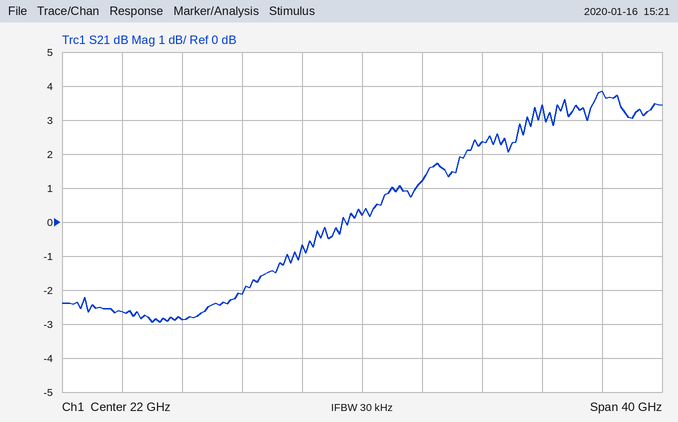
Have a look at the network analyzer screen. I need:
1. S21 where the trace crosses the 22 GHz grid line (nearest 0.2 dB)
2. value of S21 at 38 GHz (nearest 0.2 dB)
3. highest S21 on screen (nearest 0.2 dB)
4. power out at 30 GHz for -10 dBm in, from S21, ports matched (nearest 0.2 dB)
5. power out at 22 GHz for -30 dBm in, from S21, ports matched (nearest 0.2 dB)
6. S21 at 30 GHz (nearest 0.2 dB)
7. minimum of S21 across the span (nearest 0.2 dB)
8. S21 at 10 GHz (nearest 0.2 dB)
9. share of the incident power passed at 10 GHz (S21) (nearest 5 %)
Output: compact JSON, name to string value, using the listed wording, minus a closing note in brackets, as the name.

{"S21 where the trace crosses the 22 GHz grid line": "0.2 dB", "value of S21 at 38 GHz": "3.8 dB", "highest S21 on screen": "3.8 dB", "power out at 30 GHz for -10 dBm in, from S21, ports matched": "-7.6 dBm", "power out at 22 GHz for -30 dBm in, from S21, ports matched": "-29.8 dBm", "S21 at 30 GHz": "2.4 dB", "minimum of S21 across the span": "-3.0 dB", "S21 at 10 GHz": "-2.8 dB", "share of the incident power passed at 10 GHz (S21)": "50 %"}
